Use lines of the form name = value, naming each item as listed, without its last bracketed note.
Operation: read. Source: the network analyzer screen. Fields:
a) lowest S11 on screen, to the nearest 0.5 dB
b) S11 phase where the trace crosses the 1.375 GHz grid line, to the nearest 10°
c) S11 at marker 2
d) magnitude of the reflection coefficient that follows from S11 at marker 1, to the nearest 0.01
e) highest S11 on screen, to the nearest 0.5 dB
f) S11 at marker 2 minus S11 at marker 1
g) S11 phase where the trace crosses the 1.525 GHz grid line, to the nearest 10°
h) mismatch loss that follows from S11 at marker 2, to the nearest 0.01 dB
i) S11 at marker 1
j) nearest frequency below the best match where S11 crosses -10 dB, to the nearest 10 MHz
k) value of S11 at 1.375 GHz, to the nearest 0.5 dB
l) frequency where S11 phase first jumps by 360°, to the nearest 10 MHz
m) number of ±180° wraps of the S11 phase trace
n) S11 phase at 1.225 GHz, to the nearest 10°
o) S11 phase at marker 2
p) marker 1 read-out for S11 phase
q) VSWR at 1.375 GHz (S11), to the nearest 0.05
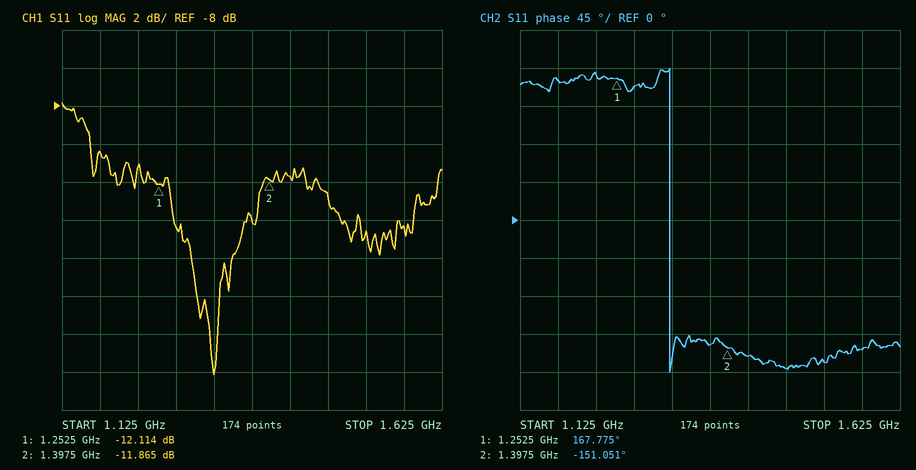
lowest S11 on screen, to the nearest 0.5 dB = -22.0 dB
S11 phase where the trace crosses the 1.375 GHz grid line, to the nearest 10° = -150°
S11 at marker 2 = -11.865 dB
magnitude of the reflection coefficient that follows from S11 at marker 1, to the nearest 0.01 = 0.25
highest S11 on screen, to the nearest 0.5 dB = -8.0 dB
S11 at marker 2 minus S11 at marker 1 = 0.249 dB
S11 phase where the trace crosses the 1.525 GHz grid line, to the nearest 10° = -170°
mismatch loss that follows from S11 at marker 2, to the nearest 0.01 dB = 0.29 dB
S11 at marker 1 = -12.114 dB
nearest frequency below the best match where S11 crosses -10 dB, to the nearest 10 MHz = 1.16 GHz
value of S11 at 1.375 GHz, to the nearest 0.5 dB = -14.0 dB
frequency where S11 phase first jumps by 360°, to the nearest 10 MHz = 1.32 GHz
number of ±180° wraps of the S11 phase trace = 1
S11 phase at 1.225 GHz, to the nearest 10° = 170°
S11 phase at marker 2 = -151.051°
marker 1 read-out for S11 phase = 167.775°
VSWR at 1.375 GHz (S11), to the nearest 0.05 = 1.50
